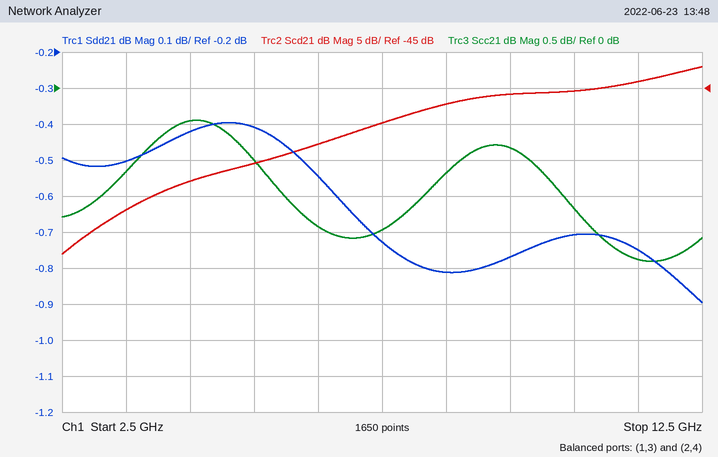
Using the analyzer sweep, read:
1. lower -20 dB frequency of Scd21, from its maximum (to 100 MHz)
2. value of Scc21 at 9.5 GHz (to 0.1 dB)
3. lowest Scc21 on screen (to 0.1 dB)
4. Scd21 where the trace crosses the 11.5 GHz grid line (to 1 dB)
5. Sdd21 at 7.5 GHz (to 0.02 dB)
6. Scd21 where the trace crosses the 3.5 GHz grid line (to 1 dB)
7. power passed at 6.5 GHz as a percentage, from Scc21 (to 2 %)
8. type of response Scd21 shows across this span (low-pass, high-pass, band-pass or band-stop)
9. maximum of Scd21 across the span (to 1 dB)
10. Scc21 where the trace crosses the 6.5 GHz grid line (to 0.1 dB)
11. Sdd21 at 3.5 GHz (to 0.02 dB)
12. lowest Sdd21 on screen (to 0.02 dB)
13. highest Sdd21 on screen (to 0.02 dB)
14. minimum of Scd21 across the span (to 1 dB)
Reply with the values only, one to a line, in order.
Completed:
3.5 GHz
-0.8 dB
-2.4 dB
-44 dB
-0.72 dB
-62 dB
64 %
high-pass
-42 dB
-1.9 dB
-0.50 dB
-0.90 dB
-0.40 dB
-68 dB
